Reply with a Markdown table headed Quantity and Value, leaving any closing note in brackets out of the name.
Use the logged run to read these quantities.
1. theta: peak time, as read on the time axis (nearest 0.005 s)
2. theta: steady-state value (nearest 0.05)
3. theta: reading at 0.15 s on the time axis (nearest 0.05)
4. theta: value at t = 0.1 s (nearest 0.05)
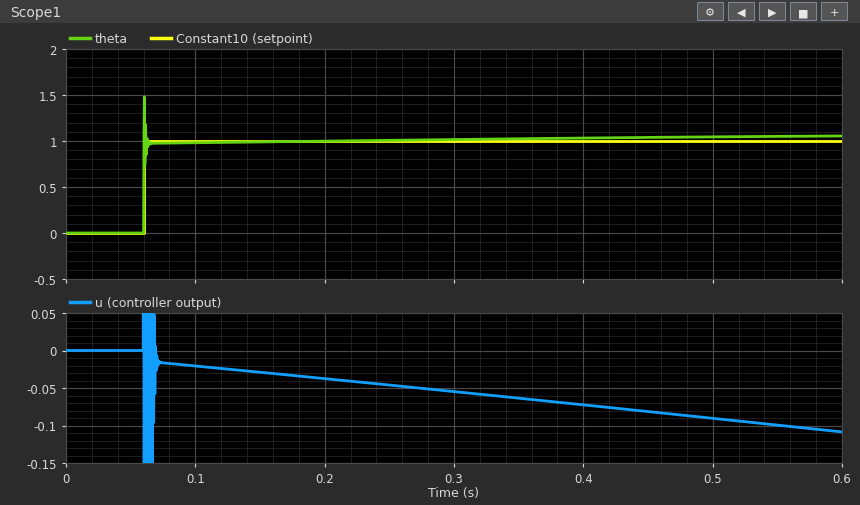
| Quantity | Value |
|---|---|
| theta: peak time, as read on the time axis | 0.060 s |
| theta: steady-state value | 1.05 |
| theta: reading at 0.15 s on the time axis | 1.00 |
| theta: value at t = 0.1 s | 1.00 |
